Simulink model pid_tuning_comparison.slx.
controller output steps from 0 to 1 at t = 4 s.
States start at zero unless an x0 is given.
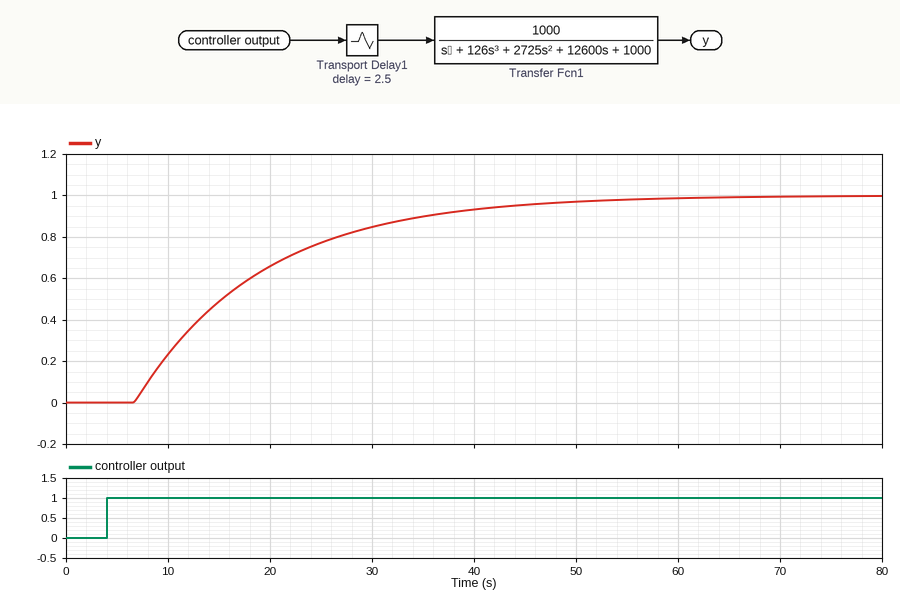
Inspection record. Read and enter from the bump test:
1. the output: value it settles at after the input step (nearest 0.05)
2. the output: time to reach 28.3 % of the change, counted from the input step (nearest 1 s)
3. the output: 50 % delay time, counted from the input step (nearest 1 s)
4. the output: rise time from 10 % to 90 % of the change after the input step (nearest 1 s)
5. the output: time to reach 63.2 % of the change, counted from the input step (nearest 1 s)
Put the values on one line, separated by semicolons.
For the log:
1.00; 7 s; 11 s; 27 s; 15 s
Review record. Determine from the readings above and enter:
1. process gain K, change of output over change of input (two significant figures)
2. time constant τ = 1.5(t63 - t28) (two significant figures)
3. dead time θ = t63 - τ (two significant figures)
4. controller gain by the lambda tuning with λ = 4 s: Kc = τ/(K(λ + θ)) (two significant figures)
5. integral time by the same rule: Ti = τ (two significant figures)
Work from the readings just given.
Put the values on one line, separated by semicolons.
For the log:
1.0; 12 s; 3.0 s; 1.7; 12 s
